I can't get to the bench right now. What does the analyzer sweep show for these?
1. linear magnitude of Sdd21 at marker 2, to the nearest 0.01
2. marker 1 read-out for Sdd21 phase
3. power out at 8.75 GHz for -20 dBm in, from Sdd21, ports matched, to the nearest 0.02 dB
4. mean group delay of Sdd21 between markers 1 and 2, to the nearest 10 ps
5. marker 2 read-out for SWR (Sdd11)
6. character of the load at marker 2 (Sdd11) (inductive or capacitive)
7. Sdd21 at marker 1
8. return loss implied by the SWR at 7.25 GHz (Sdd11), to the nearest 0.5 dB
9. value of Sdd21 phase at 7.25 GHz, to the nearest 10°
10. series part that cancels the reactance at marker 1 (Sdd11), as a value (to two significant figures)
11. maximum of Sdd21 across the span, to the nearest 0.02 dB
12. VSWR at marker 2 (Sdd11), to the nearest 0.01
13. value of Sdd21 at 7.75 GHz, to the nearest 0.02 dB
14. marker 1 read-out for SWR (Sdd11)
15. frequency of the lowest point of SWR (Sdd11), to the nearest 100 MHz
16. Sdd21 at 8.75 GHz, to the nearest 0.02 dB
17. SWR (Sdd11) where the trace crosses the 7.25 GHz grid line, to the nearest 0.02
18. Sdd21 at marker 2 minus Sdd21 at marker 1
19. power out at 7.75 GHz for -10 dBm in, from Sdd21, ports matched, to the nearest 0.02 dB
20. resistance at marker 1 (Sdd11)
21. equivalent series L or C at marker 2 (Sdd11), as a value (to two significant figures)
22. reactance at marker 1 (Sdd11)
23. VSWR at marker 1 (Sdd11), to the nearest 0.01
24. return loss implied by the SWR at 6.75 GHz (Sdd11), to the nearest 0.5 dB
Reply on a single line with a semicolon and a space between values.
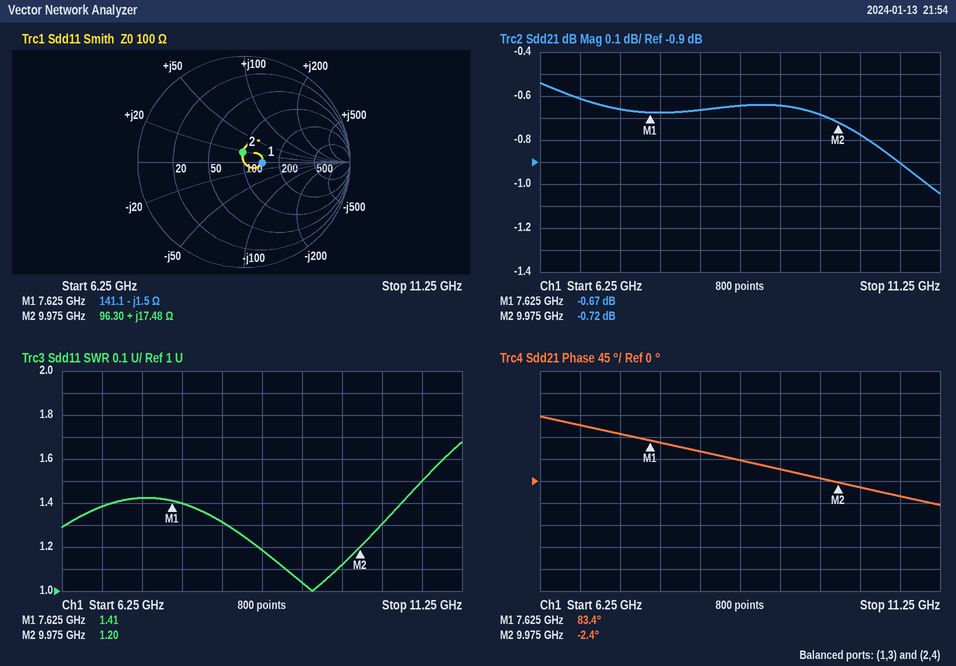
0.92; 83.4°; -20.64 dBm; 100 ps; 1.20; inductive; -0.67 dB; 15.0 dB; 100°; 31 pH; -0.54 dB; 1.20; -0.68 dB; 1.41; 9.4 GHz; -0.64 dB; 1.42; -0.05 dB; -10.68 dBm; 141.1 Ω; 280 pH; -1.5 Ω; 1.41; 16.0 dB
